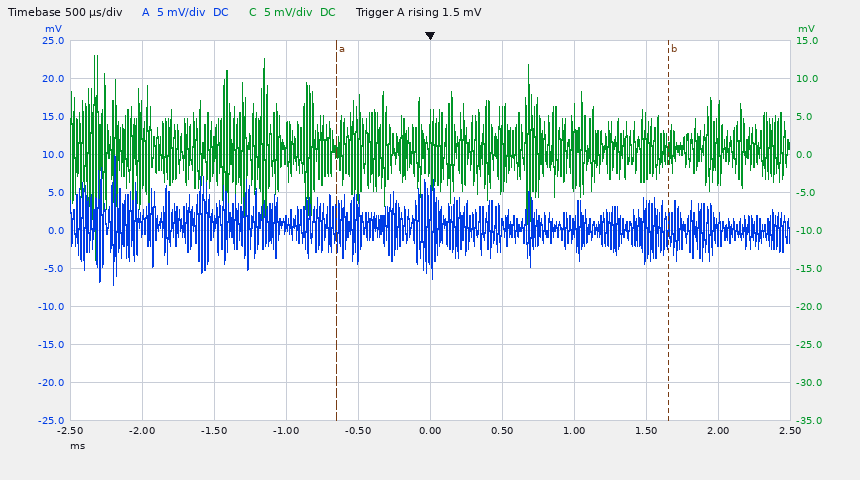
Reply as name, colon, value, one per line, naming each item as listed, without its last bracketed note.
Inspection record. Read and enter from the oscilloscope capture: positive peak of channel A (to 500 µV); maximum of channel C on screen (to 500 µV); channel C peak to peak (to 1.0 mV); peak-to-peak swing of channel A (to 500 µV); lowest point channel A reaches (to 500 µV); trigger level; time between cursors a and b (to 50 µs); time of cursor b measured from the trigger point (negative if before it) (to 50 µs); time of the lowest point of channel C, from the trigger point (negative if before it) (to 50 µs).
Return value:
positive peak of channel A: 10.0 mV
maximum of channel C on screen: 13.0 mV
channel C peak to peak: 27.0 mV
peak-to-peak swing of channel A: 17.0 mV
lowest point channel A reaches: -7.0 mV
trigger level: 1.5 mV
time between cursors a and b: 2.30 ms
time of cursor b measured from the trigger point (negative if before it): +1.65 ms
time of the lowest point of channel C, from the trigger point (negative if before it): -2.30 ms
